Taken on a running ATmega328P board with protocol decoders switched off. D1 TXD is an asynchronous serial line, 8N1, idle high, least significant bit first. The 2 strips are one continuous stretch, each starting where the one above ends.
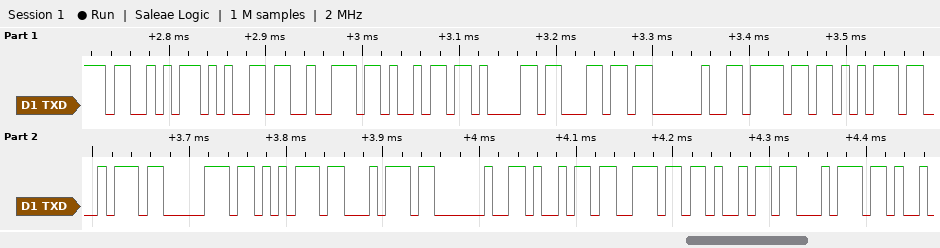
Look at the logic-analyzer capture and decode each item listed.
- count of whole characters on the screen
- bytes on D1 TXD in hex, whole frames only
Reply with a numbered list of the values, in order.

1. 18
2. 0x53 0x65 0x72 0x69 0x61 0x6C 0x20 0x6F 0x75 0x74 0x70 0x75 0x74 0x20 0x69 0x6E 0x69 0x74
